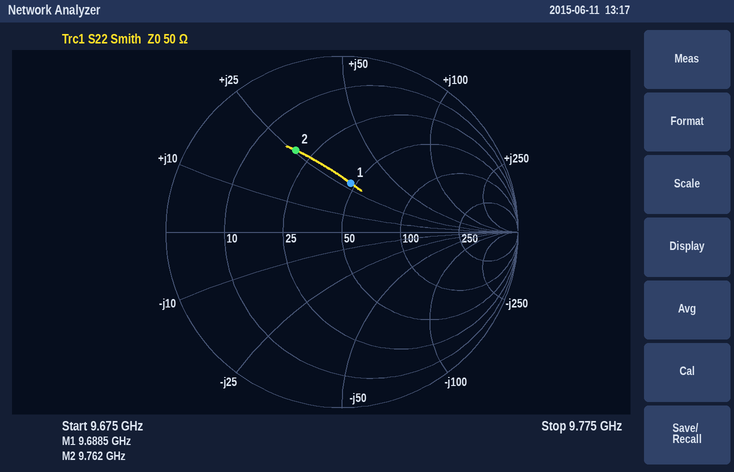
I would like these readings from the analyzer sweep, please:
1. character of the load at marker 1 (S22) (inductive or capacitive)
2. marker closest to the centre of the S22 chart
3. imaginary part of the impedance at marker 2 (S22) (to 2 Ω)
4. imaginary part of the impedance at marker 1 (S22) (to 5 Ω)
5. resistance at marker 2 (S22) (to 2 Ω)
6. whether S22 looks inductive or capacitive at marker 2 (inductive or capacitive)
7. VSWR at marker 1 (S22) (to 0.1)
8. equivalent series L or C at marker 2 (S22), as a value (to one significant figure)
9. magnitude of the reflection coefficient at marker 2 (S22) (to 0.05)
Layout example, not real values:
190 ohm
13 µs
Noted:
inductive
marker 1
+26 Ω
+30 Ω
20 Ω
inductive
1.8
400 pH
0.55
